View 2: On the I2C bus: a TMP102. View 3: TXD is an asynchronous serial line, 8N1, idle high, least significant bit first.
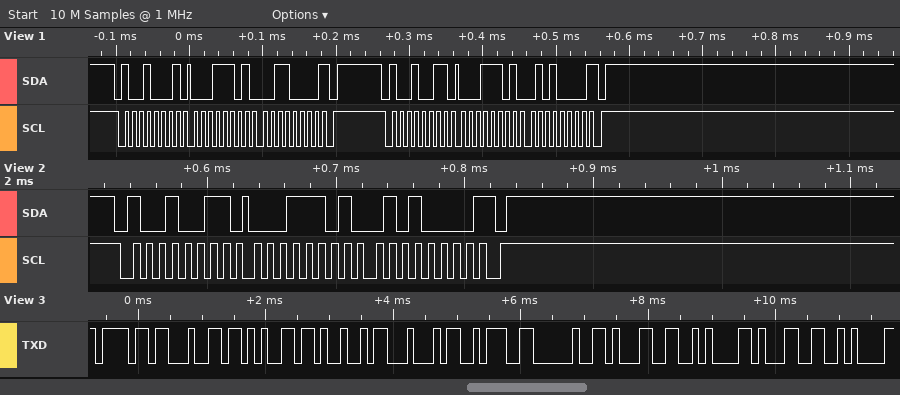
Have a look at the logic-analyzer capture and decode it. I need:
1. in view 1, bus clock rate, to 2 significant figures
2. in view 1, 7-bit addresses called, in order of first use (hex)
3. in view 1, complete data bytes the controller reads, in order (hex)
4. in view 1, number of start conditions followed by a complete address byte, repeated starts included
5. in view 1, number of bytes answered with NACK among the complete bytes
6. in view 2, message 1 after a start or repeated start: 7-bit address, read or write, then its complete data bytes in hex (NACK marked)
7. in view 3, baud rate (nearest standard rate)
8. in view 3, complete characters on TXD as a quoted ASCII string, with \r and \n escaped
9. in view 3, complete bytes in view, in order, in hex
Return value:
100 kHz
0x48 0x49
1D 30 1D 50
2
2
0x49 read: 1D 50 NACK
9600 baud
"odeID: 1\n1\n"
0x6F 0x64 0x65 0x49 0x44 0x3A 0x20 0x31 0x0A 0x31 0x0A
